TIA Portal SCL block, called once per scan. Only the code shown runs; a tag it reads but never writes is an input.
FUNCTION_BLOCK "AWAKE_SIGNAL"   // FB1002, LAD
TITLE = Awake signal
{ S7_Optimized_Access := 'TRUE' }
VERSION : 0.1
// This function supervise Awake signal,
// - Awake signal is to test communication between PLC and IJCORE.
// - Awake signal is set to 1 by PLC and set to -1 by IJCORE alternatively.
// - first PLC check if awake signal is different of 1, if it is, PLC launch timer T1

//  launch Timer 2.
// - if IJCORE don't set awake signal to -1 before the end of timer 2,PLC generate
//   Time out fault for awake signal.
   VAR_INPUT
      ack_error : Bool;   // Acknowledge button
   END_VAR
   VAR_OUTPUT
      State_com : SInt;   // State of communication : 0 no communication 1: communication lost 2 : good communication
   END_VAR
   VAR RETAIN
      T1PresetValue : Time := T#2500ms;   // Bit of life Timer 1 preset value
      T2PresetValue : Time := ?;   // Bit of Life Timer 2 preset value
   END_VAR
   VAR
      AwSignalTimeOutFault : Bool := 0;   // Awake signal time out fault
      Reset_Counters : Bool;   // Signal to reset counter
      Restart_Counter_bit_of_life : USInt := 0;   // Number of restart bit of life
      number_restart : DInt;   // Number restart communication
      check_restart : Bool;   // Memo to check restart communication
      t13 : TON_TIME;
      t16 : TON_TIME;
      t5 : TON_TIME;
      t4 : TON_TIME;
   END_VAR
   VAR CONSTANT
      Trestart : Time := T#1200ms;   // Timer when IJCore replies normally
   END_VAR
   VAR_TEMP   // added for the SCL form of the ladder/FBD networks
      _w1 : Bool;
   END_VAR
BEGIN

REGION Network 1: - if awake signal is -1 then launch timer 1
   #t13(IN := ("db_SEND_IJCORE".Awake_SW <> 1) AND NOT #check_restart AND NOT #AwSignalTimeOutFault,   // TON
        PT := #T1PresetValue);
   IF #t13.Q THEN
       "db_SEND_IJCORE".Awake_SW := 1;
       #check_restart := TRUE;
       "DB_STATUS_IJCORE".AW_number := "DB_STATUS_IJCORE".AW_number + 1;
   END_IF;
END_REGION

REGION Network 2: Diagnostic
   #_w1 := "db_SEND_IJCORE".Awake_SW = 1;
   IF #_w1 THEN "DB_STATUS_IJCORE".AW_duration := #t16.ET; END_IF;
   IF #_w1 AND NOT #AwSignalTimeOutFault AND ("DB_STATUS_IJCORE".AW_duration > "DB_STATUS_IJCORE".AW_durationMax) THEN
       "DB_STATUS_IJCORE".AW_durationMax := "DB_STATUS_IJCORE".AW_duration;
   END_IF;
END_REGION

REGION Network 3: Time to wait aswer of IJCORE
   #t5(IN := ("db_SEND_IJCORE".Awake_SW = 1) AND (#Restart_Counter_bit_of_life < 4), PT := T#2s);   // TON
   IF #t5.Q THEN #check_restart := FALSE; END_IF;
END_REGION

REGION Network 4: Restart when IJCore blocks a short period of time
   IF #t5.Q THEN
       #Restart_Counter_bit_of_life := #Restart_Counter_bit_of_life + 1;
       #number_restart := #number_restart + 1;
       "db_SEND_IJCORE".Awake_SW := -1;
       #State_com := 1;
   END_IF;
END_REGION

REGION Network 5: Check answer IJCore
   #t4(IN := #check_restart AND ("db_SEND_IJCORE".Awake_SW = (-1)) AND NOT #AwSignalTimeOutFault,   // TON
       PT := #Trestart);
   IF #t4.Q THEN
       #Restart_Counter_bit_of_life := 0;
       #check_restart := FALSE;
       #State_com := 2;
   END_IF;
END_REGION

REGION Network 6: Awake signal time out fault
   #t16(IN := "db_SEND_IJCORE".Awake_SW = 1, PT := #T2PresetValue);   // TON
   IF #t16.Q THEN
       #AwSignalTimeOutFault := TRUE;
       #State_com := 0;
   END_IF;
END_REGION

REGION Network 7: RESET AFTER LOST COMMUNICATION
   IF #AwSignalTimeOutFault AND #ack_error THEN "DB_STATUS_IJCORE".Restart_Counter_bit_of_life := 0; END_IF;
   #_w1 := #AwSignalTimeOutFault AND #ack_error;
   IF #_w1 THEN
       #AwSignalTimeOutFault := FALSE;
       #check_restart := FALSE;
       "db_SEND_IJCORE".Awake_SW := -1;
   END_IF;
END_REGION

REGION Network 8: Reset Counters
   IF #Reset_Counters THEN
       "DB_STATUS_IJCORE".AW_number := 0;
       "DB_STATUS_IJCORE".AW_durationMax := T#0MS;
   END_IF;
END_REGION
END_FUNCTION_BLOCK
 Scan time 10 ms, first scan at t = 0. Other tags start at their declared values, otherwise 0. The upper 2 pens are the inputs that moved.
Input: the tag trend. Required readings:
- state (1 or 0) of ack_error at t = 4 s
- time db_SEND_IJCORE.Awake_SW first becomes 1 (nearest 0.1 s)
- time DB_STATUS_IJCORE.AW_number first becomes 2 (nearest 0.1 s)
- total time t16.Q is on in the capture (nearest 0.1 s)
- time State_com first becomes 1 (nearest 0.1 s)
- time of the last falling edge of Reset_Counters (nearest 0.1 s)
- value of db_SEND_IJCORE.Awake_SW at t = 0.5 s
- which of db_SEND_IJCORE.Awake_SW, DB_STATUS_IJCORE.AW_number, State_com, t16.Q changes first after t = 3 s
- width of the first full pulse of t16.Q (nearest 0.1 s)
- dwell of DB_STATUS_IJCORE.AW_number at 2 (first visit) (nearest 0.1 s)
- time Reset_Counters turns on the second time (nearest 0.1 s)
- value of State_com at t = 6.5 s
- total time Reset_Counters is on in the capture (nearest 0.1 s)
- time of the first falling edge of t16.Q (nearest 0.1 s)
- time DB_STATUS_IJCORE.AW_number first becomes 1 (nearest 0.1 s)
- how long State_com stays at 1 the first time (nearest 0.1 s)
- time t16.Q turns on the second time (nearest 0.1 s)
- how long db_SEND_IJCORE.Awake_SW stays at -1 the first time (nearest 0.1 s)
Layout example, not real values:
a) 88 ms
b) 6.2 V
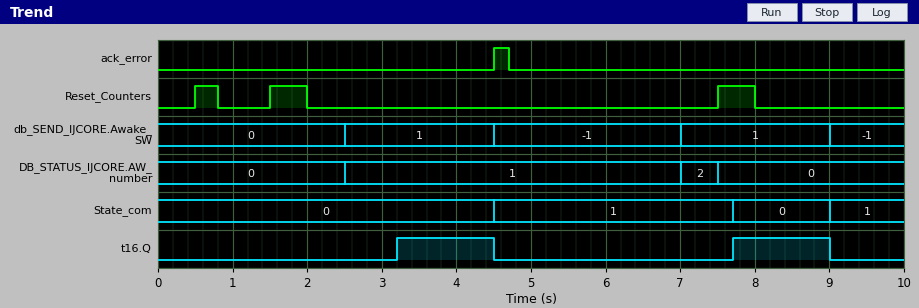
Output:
a) 0
b) 2.5 s
c) 7.0 s
d) 2.6 s
e) 4.5 s
f) 8.0 s
g) 0
h) t16.Q
i) 1.3 s
j) 0.5 s
k) 1.5 s
l) 1
m) 1.3 s
n) 4.5 s
o) 2.5 s
p) 3.2 s
q) 7.7 s
r) 2.5 s
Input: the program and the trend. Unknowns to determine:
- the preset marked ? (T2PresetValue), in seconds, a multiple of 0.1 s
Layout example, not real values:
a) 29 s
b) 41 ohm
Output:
a) 0.7 s
